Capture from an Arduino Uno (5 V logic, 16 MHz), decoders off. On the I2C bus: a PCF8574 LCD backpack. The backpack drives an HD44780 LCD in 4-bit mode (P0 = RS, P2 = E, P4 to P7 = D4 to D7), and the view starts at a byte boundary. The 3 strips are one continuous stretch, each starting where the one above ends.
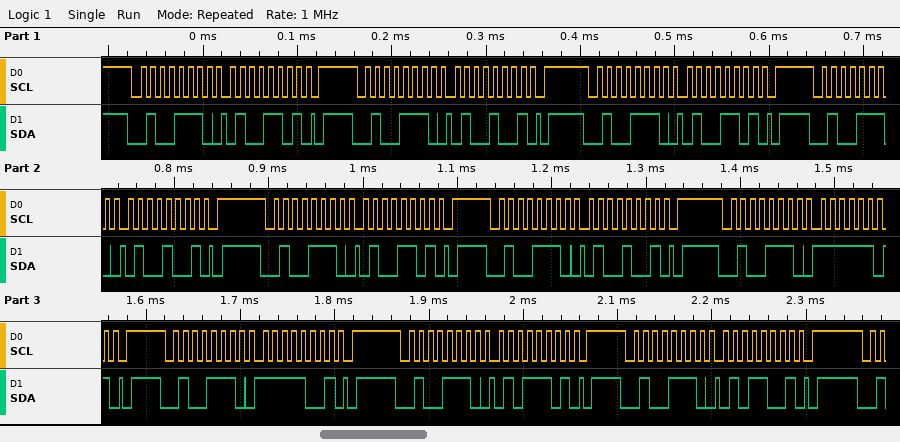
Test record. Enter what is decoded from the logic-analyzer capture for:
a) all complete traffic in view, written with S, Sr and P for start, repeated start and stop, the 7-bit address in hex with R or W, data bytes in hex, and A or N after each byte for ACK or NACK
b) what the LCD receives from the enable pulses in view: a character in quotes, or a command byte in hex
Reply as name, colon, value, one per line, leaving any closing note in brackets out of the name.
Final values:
all complete traffic in view, written with S, Sr and P for start, repeated start and stop, the 7-bit address in hex with R or W, data bytes in hex, and A or N after each byte for ACK or NACK: S 27W A 4D A P S 27W A 49 A P S 27W A 4D A P S 27W A 49 A P S 27W A 4D A P S 27W A 49 A P S 27W A FD A P S 27W A F9 A P S 27W A 5D A P S 27W A 59 A P
what the LCD receives from the enable pulses in view: a character in quotes, or a command byte in hex: 'D' 'O'
